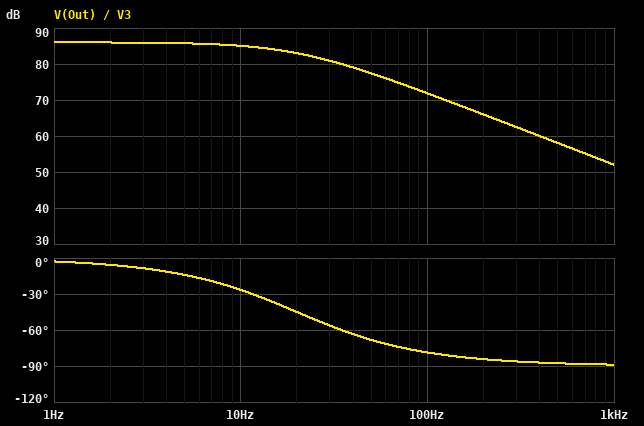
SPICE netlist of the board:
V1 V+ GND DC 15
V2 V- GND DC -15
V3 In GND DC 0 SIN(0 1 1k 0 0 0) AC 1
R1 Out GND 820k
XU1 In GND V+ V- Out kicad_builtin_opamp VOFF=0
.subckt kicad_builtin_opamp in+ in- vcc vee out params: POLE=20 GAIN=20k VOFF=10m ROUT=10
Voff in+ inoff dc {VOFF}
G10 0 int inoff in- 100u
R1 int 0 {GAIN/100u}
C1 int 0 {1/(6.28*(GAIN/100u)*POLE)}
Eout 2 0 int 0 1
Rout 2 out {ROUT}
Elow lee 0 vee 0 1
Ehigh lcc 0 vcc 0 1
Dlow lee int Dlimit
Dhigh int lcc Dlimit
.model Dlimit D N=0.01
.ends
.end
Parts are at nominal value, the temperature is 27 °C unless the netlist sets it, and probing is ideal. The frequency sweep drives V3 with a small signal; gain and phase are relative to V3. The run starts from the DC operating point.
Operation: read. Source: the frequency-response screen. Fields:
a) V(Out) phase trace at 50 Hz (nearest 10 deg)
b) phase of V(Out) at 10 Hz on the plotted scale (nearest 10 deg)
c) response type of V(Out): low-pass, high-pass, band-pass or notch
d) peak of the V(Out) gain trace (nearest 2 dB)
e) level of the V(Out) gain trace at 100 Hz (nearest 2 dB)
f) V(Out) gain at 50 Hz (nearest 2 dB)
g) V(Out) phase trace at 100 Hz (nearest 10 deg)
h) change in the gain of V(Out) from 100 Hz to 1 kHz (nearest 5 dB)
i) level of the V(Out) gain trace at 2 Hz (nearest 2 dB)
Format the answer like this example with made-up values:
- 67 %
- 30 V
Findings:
- -70 deg
- -30 deg
- low-pass
- 86 dB
- 72 dB
- 78 dB
- -80 deg
- -20 dB
- 86 dB
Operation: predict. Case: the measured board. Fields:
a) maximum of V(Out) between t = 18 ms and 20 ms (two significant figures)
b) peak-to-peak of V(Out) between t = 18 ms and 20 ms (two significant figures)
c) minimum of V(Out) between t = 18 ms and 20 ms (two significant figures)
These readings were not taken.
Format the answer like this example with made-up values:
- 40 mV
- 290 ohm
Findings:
- 15 V
- 30 V
- -15 V
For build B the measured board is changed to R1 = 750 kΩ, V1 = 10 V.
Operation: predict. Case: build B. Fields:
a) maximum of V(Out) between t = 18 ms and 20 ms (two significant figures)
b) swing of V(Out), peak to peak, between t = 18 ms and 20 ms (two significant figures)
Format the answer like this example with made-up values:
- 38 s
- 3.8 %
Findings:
- 10 V
- 25 V
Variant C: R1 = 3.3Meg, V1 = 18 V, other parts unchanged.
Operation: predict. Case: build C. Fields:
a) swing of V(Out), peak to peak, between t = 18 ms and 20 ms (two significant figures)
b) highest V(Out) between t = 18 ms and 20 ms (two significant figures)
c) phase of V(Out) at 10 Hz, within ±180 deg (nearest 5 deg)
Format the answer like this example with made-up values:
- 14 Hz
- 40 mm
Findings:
- 33 V
- 18 V
- -25 deg
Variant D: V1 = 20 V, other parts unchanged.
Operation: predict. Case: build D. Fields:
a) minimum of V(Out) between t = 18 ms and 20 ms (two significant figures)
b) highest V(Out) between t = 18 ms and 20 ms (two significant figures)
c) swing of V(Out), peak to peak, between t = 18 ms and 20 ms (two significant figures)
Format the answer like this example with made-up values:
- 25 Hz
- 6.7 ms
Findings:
- -15 V
- 20 V
- 35 V
